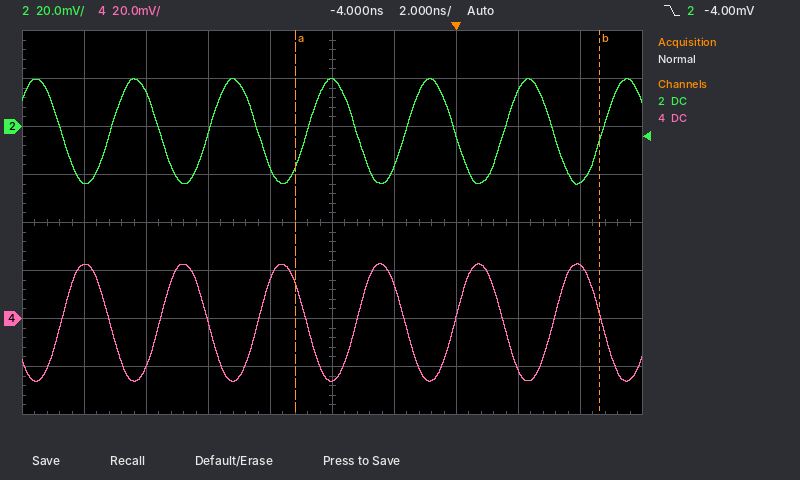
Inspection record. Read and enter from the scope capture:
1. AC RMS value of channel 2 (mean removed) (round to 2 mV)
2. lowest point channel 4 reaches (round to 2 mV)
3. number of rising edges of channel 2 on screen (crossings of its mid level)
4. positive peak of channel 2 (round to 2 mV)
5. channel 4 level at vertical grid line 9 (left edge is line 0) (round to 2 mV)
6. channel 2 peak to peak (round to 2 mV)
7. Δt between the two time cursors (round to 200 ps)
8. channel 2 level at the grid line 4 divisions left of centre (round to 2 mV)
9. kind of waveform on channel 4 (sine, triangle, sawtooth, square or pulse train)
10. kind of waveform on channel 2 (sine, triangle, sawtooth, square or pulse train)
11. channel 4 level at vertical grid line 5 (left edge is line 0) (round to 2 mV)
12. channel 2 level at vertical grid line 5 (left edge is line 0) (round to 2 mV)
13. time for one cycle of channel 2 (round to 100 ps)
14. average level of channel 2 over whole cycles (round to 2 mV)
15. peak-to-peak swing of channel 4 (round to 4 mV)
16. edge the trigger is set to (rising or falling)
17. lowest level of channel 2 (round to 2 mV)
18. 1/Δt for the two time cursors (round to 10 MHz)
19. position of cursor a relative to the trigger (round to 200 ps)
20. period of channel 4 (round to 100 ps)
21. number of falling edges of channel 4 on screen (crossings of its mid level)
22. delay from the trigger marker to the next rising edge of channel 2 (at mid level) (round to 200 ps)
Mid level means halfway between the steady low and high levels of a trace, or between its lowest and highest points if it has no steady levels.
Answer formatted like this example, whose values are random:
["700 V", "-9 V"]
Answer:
["16 mV", "-26 mV", "6", "20 mV", "22 mV", "44 mV", "9.8 ns", "-24 mV", "sine", "sine", "-26 mV", "20 mV", "3.2 ns", "-2 mV", "48 mV", "falling", "-24 mV", "100 MHz", "-5.2 ns", "3.2 ns", "6", "1.6 ns"]
